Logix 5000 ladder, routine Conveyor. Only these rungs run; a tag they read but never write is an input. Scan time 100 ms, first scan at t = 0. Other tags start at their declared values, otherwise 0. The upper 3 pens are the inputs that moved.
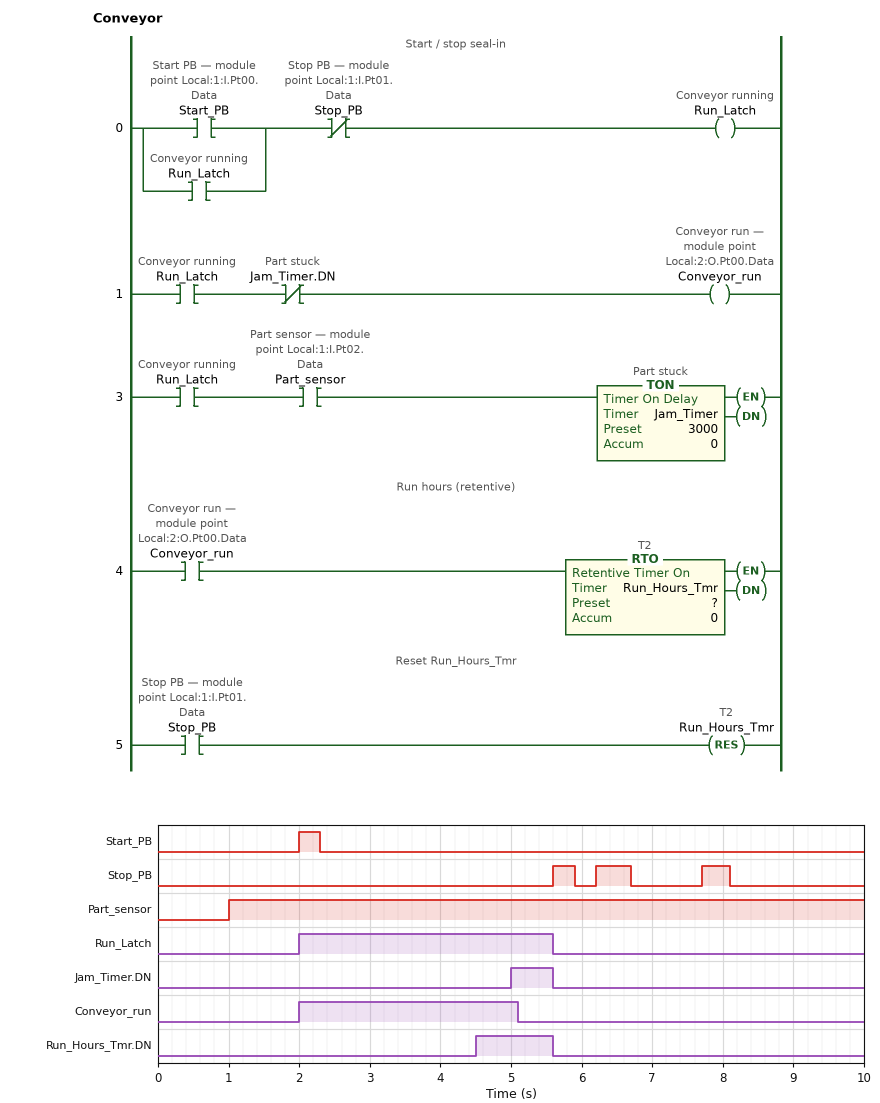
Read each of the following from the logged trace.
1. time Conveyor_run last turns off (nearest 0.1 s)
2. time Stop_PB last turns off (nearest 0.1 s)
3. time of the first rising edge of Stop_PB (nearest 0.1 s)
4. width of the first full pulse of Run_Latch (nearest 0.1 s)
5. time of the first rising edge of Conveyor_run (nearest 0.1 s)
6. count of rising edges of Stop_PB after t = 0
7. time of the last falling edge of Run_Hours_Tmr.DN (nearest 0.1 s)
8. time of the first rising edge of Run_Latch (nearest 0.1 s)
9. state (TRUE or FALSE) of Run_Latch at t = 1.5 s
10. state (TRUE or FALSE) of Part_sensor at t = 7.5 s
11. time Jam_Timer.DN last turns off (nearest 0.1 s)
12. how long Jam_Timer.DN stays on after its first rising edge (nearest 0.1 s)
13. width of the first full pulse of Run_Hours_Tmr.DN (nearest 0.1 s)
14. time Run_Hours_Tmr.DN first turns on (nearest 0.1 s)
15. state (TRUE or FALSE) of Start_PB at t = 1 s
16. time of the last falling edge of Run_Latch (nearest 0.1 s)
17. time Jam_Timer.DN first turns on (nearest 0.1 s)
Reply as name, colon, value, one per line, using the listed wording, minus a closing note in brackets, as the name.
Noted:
time Conveyor_run last turns off: 5.1 s
time Stop_PB last turns off: 8.1 s
time of the first rising edge of Stop_PB: 5.6 s
width of the first full pulse of Run_Latch: 3.6 s
time of the first rising edge of Conveyor_run: 2.0 s
count of rising edges of Stop_PB after t = 0: 3
time of the last falling edge of Run_Hours_Tmr.DN: 5.6 s
time of the first rising edge of Run_Latch: 2.0 s
state (TRUE or FALSE) of Run_Latch at t = 1.5 s: FALSE
state (TRUE or FALSE) of Part_sensor at t = 7.5 s: TRUE
time Jam_Timer.DN last turns off: 5.6 s
how long Jam_Timer.DN stays on after its first rising edge: 0.6 s
width of the first full pulse of Run_Hours_Tmr.DN: 1.1 s
time Run_Hours_Tmr.DN first turns on: 4.5 s
state (TRUE or FALSE) of Start_PB at t = 1 s: FALSE
time of the last falling edge of Run_Latch: 5.6 s
time Jam_Timer.DN first turns on: 5.0 s
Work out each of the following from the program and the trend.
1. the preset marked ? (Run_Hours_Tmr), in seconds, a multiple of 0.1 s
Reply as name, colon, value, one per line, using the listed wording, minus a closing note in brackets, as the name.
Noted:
the preset marked ? (Run_Hours_Tmr), in seconds, a multiple of 0.1 s: 2.5 s
